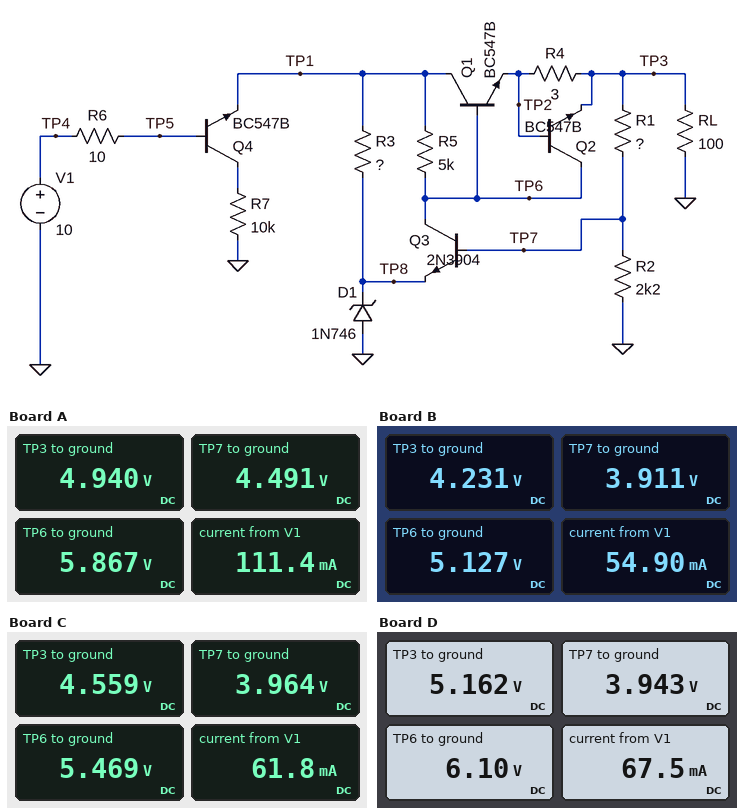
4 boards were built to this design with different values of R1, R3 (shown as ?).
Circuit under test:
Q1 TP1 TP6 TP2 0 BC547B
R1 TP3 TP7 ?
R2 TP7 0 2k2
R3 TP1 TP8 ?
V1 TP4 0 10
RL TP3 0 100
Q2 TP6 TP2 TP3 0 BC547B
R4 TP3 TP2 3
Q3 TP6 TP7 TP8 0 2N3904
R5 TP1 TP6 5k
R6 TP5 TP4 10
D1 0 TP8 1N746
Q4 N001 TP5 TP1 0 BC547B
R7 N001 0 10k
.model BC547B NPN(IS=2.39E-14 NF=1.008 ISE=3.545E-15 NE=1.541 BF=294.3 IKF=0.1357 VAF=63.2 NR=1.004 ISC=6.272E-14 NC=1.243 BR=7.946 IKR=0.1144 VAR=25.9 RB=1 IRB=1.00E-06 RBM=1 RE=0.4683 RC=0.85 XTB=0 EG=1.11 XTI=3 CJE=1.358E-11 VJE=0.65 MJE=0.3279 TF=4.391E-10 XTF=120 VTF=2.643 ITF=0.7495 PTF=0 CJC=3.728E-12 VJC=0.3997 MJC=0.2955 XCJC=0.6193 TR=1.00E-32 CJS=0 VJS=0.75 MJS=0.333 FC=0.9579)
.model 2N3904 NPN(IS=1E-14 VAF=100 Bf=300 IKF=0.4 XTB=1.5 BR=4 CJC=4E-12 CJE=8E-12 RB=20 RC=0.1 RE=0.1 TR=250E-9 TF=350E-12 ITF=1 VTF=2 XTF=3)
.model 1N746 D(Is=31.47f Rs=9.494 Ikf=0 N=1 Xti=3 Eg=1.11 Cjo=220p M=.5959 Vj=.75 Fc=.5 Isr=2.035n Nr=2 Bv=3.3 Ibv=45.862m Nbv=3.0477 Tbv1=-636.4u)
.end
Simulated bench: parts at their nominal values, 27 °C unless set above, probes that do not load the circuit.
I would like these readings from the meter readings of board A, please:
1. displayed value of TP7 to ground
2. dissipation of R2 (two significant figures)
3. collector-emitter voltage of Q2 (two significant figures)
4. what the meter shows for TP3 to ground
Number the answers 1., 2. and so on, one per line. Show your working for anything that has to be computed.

1. 4.491 V
2. (4.491 V)^2 / 2.2 kΩ = 9.2 mW
3. 5.867 V - 4.94 V = 930 mV
4. 4.940 V
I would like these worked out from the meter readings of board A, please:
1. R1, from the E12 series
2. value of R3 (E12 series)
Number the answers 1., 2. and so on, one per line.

1. 220 Ω
2. 68 Ω
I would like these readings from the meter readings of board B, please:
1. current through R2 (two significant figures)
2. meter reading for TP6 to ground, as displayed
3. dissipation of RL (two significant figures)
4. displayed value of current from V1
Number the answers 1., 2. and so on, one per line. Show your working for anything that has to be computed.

1. (3.911 V) / 2.2 kΩ = 1.8 mA
2. 5.127 V
3. (4.231 V)^2 / 100 Ω = 180 mW
4. 54.90 mA
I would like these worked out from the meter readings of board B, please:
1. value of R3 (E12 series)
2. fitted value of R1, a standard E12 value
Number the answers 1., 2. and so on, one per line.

1. 560 Ω
2. 180 Ω
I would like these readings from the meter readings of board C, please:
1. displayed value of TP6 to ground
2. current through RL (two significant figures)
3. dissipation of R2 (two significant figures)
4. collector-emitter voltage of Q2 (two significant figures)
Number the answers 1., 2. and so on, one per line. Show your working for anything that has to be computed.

1. 5.469 V
2. (4.559 V) / 100 Ω = 46 mA
3. (3.964 V)^2 / 2.2 kΩ = 7.1 mW
4. 5.469 V - 4.559 V = 910 mV
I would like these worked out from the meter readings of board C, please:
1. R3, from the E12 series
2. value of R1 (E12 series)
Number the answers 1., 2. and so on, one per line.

1. 390 Ω
2. 330 Ω
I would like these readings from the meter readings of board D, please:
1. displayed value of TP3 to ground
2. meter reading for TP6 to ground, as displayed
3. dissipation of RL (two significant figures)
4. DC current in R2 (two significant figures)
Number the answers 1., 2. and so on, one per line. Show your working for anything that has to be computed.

1. 5.162 V
2. 6.10 V
3. (5.162 V)^2 / 100 Ω = 270 mW
4. (3.943 V) / 2.2 kΩ = 1.8 mA
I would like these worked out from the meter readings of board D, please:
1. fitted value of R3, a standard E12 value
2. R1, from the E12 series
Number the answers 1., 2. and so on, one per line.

1. 390 Ω
2. 680 Ω
